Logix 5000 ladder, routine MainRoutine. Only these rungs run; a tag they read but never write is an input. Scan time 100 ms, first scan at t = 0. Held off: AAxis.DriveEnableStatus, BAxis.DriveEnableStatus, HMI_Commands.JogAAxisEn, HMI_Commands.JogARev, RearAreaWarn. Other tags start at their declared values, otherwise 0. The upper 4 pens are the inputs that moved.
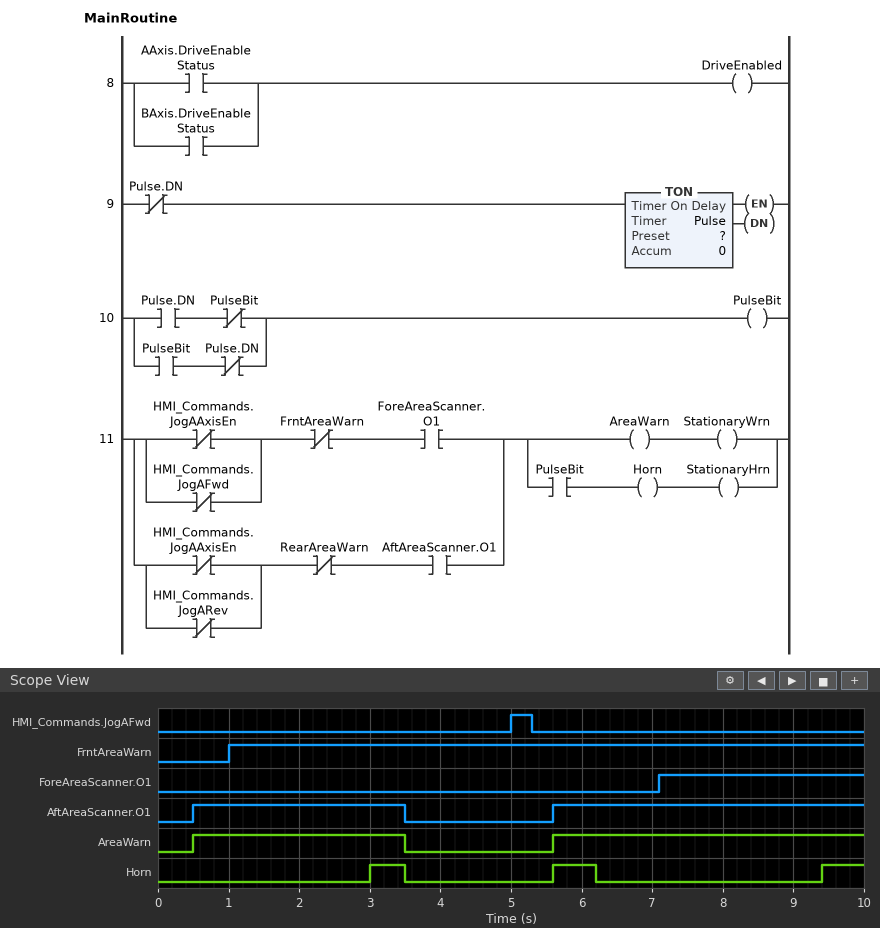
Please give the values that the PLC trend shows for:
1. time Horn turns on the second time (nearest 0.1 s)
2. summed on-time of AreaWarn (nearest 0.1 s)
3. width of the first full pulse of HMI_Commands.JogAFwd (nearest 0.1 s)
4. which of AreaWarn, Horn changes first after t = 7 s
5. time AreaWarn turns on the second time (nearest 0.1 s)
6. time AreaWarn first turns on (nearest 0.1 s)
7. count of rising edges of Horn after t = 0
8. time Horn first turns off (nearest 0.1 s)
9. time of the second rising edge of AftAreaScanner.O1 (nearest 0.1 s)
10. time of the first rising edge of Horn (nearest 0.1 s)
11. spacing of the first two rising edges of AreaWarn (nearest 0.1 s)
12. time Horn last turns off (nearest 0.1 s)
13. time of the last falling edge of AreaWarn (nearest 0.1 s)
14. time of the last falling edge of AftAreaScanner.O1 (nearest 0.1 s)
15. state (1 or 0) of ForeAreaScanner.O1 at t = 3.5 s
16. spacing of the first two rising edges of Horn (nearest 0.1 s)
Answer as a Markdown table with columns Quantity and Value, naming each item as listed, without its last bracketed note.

| Quantity | Value |
|---|---|
| time Horn turns on the second time | 5.6 s |
| summed on-time of AreaWarn | 7.4 s |
| width of the first full pulse of HMI_Commands.JogAFwd | 0.3 s |
| which of AreaWarn, Horn changes first after t = 7 s | Horn |
| time AreaWarn turns on the second time | 5.6 s |
| time AreaWarn first turns on | 0.5 s |
| count of rising edges of Horn after t = 0 | 3 |
| time Horn first turns off | 3.5 s |
| time of the second rising edge of AftAreaScanner.O1 | 5.6 s |
| time of the first rising edge of Horn | 3.0 s |
| spacing of the first two rising edges of AreaWarn | 5.1 s |
| time Horn last turns off | 6.2 s |
| time of the last falling edge of AreaWarn | 3.5 s |
| time of the last falling edge of AftAreaScanner.O1 | 3.5 s |
| state (1 or 0) of ForeAreaScanner.O1 at t = 3.5 s | 0 |
| spacing of the first two rising edges of Horn | 2.6 s |
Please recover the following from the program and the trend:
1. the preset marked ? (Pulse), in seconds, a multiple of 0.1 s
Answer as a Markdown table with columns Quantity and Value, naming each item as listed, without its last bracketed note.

| Quantity | Value |
|---|---|
| the preset marked ? (Pulse), in seconds, a multiple of 0.1 s | 3.0 s |
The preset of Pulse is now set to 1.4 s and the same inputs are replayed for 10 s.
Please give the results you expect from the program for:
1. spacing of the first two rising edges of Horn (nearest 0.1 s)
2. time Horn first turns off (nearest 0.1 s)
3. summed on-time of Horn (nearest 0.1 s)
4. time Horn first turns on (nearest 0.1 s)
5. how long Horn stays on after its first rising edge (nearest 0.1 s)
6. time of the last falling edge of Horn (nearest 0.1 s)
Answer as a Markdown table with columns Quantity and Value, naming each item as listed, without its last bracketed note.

| Quantity | Value |
|---|---|
| spacing of the first two rising edges of Horn | 4.2 s |
| time Horn first turns off | 3.0 s |
| summed on-time of Horn | 3.8 s |
| time Horn first turns on | 1.4 s |
| how long Horn stays on after its first rising edge | 1.6 s |
| time of the last falling edge of Horn | 9.4 s |
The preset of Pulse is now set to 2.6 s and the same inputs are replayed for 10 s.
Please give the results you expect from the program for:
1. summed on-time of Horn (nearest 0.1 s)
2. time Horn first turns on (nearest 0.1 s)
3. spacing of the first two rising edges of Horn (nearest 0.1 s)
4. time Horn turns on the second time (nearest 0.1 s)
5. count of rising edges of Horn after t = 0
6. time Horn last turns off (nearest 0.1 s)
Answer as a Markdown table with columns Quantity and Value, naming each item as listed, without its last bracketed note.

| Quantity | Value |
|---|---|
| summed on-time of Horn | 2.7 s |
| time Horn first turns on | 2.6 s |
| spacing of the first two rising edges of Horn | 5.6 s |
| time Horn turns on the second time | 8.2 s |
| count of rising edges of Horn after t = 0 | 2 |
| time Horn last turns off | 3.5 s |
